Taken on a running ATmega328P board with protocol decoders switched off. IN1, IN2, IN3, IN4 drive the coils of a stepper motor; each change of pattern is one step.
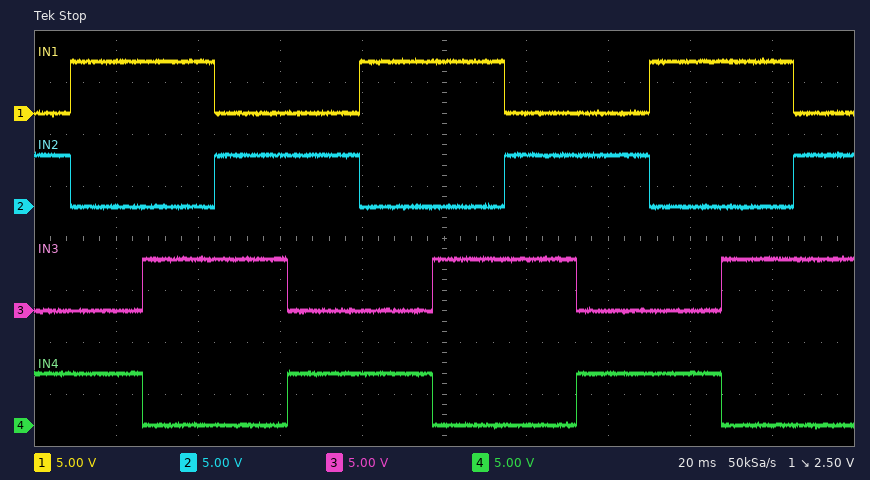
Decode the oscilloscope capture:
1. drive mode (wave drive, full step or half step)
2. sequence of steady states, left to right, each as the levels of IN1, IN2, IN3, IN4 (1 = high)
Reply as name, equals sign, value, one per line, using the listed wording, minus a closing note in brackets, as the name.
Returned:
drive mode = full step
sequence of steady states, left to right, each as the levels of IN1, IN2, IN3, IN4 = 0101 1001 1010 0110 0101 1001 1010 0110 0101 1001 1010 0110
